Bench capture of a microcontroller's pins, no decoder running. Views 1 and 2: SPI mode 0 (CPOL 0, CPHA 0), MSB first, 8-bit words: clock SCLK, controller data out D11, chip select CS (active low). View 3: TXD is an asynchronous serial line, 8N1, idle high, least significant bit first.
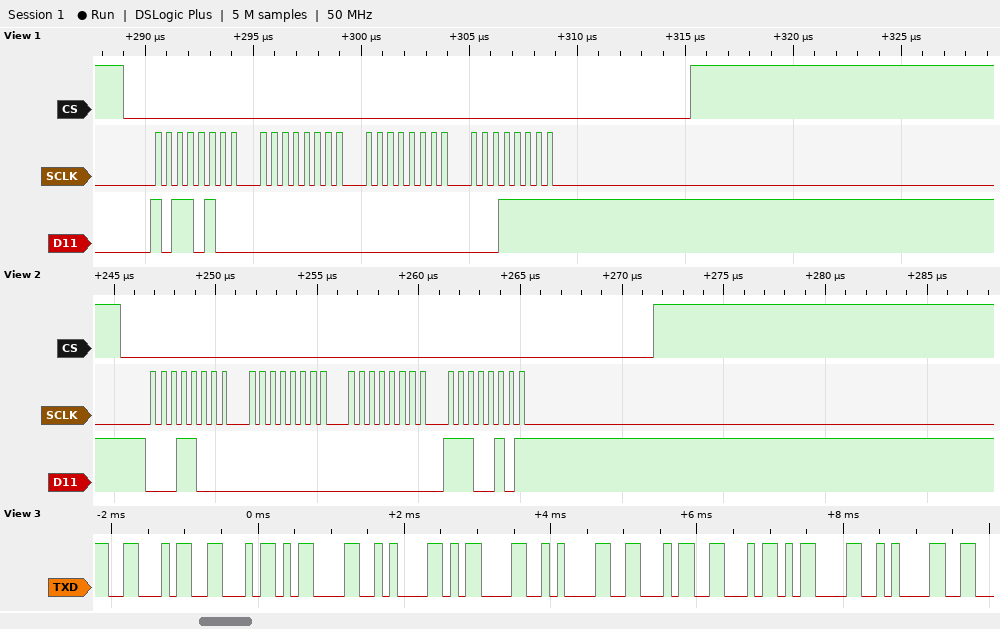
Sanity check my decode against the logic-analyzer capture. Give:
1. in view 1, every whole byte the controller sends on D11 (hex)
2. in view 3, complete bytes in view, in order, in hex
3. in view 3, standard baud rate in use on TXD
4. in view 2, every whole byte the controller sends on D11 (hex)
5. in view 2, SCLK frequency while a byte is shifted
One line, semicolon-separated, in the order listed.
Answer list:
B4 00 00 1F; 46 46 0D 0A 0D 0A 46 46 0D 0A; 9600 baud; 18 00 00 E5; 2 MHz
